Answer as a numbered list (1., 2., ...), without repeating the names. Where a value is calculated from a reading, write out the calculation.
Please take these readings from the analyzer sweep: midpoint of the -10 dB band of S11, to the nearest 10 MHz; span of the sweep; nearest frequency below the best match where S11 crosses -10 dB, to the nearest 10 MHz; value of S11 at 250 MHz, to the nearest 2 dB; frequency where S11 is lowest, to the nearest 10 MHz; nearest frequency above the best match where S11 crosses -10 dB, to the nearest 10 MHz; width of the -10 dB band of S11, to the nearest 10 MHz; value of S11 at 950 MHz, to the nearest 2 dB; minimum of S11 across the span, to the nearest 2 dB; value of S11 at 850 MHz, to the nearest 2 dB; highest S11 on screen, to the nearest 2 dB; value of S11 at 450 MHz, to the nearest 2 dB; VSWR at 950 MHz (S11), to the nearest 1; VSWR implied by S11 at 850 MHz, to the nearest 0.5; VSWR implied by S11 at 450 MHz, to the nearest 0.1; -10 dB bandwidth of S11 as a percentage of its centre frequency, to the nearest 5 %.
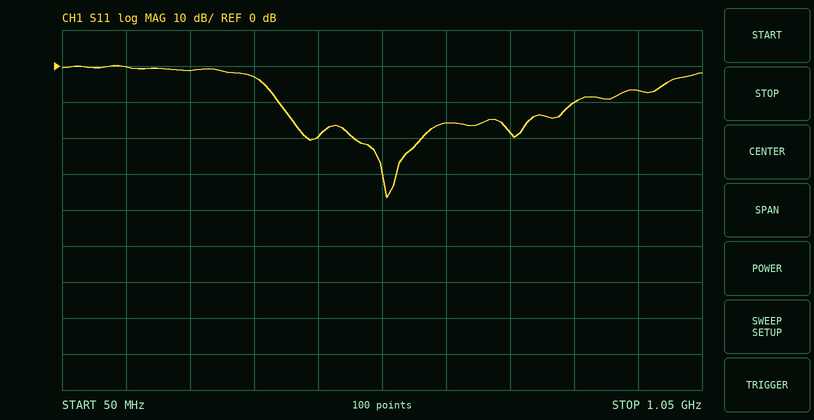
1. 620 MHz
2. 1 GHz
3. 390 MHz
4. -2 dB
5. 560 MHz
6. 850 MHz
7. 850 MHz − 390 MHz = 460 MHz
8. -6 dB
9. -36 dB
10. -10 dB
11. 0 dB
12. -20 dB
13. |Γ| = 10^(-6/20) = 0.5012; VSWR = (1 + 0.5012)/(1 − 0.5012) ≈ 3
14. |Γ| = 10^(-10/20) = 0.3162; VSWR = (1 + 0.3162)/(1 − 0.3162) ≈ 1.92, so 2.0 to the nearest 0.5
15. |Γ| = 10^(-20/20) = 0.1000; VSWR = (1 + 0.1000)/(1 − 0.1000) ≈ 1.2
16. 460 MHz / 620 MHz ≈ 74.2 %, so 75 % to the nearest 5 %
